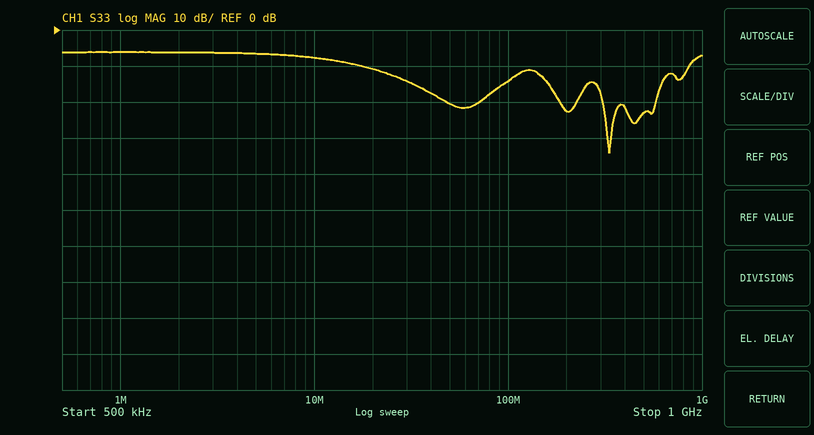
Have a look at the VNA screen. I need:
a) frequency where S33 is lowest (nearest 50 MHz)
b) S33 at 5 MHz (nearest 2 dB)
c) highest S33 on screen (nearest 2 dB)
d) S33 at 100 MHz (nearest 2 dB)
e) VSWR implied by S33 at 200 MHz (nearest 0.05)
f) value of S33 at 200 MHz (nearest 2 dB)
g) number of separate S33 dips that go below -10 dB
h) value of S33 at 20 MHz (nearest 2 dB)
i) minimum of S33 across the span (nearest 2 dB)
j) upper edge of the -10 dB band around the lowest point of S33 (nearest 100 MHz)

350 MHz
-6 dB
-6 dB
-14 dB
1.15
-22 dB
4
-10 dB
-34 dB
900 MHz
